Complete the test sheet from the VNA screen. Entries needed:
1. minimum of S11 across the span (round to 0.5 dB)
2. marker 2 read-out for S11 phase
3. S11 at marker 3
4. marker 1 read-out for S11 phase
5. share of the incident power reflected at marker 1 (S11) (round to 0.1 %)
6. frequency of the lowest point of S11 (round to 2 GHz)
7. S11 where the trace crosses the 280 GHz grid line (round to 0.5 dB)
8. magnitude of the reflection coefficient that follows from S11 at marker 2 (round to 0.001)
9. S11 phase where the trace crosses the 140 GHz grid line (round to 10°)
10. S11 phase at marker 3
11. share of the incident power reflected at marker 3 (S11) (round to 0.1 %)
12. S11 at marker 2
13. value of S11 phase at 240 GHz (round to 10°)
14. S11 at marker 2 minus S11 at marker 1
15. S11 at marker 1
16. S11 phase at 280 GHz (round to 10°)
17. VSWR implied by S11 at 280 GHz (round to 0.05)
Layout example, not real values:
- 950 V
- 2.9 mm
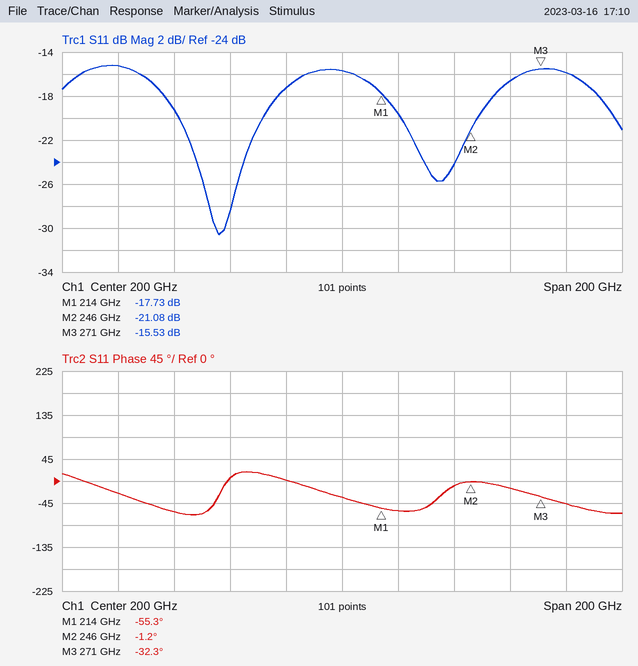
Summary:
- -30.5 dB
- -1.2°
- -15.53 dB
- -55.3°
- 1.7 %
- 156 GHz
- -16.0 dB
- 0.088
- -60°
- -32.3°
- 2.8 %
- -21.08 dB
- -10°
- -3.35 dB
- -17.73 dB
- -50°
- 1.40
